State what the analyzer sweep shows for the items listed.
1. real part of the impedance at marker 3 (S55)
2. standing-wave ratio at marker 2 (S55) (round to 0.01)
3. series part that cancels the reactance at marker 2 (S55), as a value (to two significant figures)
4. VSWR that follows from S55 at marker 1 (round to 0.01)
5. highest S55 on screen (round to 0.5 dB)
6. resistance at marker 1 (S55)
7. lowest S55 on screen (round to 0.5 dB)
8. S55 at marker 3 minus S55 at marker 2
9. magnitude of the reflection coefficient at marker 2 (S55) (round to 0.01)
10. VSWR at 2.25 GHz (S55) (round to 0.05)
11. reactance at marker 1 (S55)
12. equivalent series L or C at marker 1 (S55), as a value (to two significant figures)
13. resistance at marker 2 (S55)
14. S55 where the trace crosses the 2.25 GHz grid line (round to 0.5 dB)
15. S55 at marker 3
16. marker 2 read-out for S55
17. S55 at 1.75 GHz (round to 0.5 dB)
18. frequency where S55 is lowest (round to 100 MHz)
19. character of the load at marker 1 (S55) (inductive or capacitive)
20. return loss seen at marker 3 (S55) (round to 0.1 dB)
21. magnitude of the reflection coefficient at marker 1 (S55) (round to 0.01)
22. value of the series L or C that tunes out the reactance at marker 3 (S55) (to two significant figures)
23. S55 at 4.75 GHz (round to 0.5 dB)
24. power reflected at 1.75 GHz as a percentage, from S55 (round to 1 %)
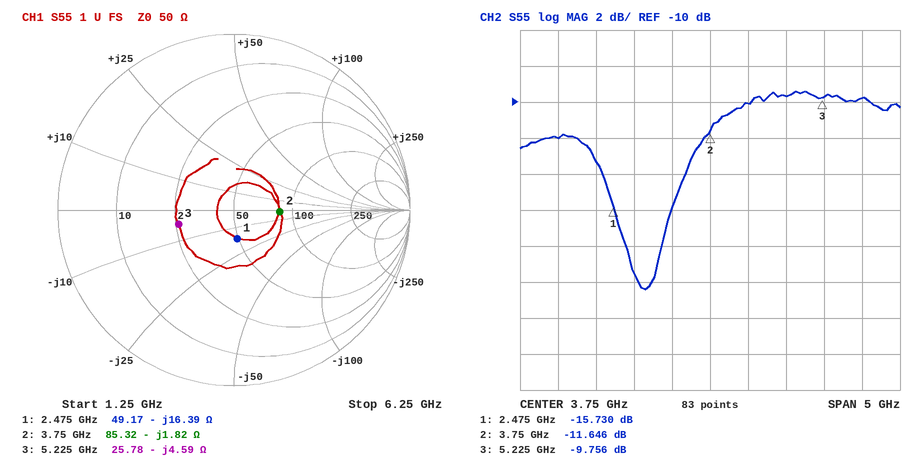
25.78 Ω
1.71
77 pH
1.39
-9.5 dB
49.17 Ω
-20.5 dB
1.890 dB
0.26
1.55
-16.39 Ω
3.9 pF
85.32 Ω
-13.5 dB
-9.756 dB
-11.646 dB
-12.0 dB
2.9 GHz
capacitive
9.8 dB
0.16
140 pH
-9.5 dB
6 %
